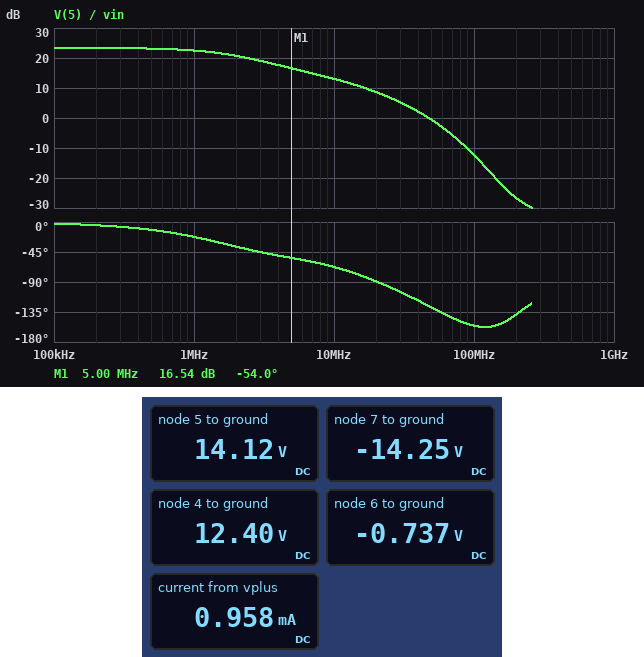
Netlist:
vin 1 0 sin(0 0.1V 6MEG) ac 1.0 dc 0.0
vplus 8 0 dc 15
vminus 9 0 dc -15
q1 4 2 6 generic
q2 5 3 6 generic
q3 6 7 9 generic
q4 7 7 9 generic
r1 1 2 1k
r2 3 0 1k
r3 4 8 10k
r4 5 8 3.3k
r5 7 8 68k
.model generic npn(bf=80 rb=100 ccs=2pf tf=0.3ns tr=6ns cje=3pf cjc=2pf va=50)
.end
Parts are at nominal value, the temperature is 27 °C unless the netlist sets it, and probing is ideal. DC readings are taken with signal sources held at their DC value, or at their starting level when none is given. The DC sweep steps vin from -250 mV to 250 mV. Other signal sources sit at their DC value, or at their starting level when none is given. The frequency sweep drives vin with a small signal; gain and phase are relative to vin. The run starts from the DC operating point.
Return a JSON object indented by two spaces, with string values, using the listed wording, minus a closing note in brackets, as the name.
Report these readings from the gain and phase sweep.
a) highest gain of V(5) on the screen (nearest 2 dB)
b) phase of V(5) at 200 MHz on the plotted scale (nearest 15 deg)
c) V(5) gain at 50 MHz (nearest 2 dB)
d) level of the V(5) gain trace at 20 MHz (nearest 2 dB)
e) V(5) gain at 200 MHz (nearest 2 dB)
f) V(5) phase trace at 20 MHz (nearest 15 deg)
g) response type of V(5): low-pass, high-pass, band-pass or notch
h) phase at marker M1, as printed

{
  "highest gain of V(5) on the screen": "24 dB",
  "phase of V(5) at 200 MHz on the plotted scale": "-135 deg",
  "V(5) gain at 50 MHz": "0 dB",
  "level of the V(5) gain trace at 20 MHz": "8 dB",
  "V(5) gain at 200 MHz": "-26 dB",
  "V(5) phase trace at 20 MHz": "-90 deg",
  "response type of V(5): low-pass, high-pass, band-pass or notch": "low-pass",
  "phase at marker M1, as printed": "-54.0 deg"
}
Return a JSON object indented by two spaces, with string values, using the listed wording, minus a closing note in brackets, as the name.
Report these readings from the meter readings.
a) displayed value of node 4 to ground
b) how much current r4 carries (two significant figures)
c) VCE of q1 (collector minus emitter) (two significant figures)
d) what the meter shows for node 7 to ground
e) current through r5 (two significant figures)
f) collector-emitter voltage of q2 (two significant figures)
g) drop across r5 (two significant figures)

{
  "displayed value of node 4 to ground": "12.40 V",
  "how much current r4 carries": "270 µA",
  "VCE of q1 (collector minus emitter)": "13 V",
  "what the meter shows for node 7 to ground": "-14.25 V",
  "current through r5": "430 µA",
  "collector-emitter voltage of q2": "15 V",
  "drop across r5": "29 V"
}
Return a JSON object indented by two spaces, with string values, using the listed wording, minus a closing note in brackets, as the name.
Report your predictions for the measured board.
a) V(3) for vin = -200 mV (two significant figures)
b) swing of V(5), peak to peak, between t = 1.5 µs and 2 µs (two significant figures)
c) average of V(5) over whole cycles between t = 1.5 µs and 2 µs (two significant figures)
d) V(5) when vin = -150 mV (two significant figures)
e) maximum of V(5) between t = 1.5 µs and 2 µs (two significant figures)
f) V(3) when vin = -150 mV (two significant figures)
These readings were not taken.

{
  "V(3) for vin = -200 mV": "-5.2 mV",
  "swing of V(5), peak to peak, between t = 1.5 µs and 2 µs": "1.1 V",
  "average of V(5) over whole cycles between t = 1.5 µs and 2 µs": "14 V",
  "V(5) when vin = -150 mV": "13 V",
  "maximum of V(5) between t = 1.5 µs and 2 µs": "15 V",
  "V(3) when vin = -150 mV": "-5.2 mV"
}
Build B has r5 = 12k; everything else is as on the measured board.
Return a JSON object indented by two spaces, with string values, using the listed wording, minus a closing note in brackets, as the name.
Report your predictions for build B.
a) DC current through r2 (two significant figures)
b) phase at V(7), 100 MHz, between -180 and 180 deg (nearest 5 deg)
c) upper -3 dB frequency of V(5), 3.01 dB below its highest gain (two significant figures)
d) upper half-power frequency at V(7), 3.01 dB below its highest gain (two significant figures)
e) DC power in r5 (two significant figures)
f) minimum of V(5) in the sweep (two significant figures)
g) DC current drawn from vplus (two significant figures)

{
  "DC current through r2": "17 µA",
  "phase at V(7), 100 MHz, between -180 and 180 deg": "15 deg",
  "upper -3 dB frequency of V(5), 3.01 dB below its highest gain": "530 kHz",
  "upper half-power frequency at V(7), 3.01 dB below its highest gain": "340 MHz",
  "DC power in r5": "71 mW",
  "minimum of V(5) in the sweep": "5.2 V",
  "DC current drawn from vplus": "5.4 mA"
}
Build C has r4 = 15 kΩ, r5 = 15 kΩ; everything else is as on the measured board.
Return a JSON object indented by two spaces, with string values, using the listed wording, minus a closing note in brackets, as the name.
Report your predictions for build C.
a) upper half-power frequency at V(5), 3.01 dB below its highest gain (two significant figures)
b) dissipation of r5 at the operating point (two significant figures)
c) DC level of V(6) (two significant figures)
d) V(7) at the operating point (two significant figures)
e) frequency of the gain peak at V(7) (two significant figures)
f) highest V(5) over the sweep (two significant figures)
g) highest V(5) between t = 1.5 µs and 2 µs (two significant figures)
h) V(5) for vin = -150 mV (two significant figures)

{
  "upper half-power frequency at V(5), 3.01 dB below its highest gain": "4.9 MHz",
  "dissipation of r5 at the operating point": "57 mW",
  "DC level of V(6)": "-800 mV",
  "V(7) at the operating point": "-14 V",
  "frequency of the gain peak at V(7)": "130 MHz",
  "highest V(5) over the sweep": "5.6 V",
  "highest V(5) between t = 1.5 µs and 2 µs": "230 mV",
  "V(5) for vin = -150 mV": "-880 mV"
}
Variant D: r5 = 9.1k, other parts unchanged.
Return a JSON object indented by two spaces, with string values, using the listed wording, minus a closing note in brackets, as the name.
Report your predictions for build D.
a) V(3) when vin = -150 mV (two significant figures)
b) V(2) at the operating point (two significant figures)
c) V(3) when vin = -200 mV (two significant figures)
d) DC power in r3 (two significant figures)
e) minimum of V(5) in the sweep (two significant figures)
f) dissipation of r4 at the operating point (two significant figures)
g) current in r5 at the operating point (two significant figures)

{
  "V(3) when vin = -150 mV": "-46 mV",
  "V(2) at the operating point": "-31 mV",
  "V(3) when vin = -200 mV": "-47 mV",
  "DC power in r3": "25 mW",
  "minimum of V(5) in the sweep": "2.1 V",
  "dissipation of r4 at the operating point": "18 mW",
  "current in r5 at the operating point": "3.2 mA"
}
